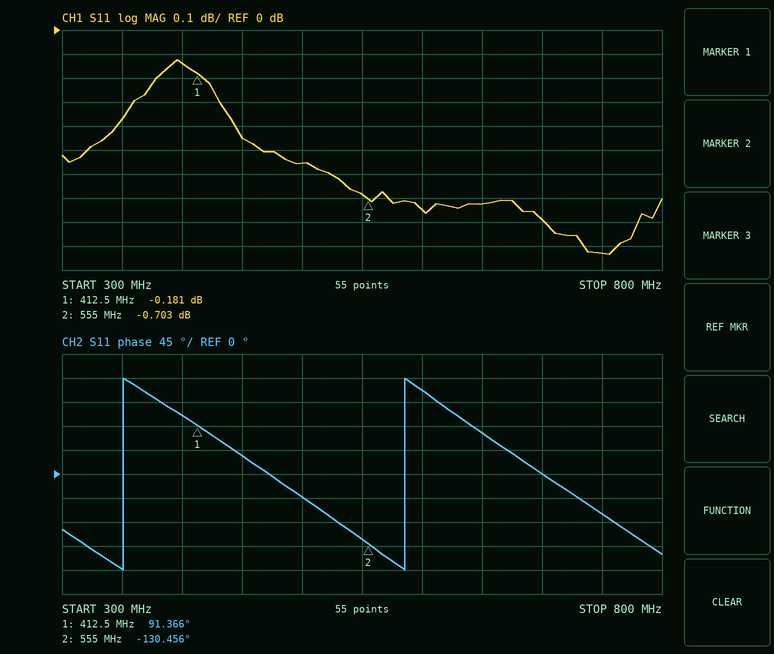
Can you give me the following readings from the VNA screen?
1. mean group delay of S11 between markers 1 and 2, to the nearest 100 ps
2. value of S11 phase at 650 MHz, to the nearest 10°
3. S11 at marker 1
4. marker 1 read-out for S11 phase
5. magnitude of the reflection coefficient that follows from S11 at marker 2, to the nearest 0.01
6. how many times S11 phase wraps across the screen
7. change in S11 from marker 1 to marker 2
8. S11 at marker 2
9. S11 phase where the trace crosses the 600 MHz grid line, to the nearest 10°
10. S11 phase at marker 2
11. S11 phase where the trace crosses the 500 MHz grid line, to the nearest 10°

4.3 ns
80°
-0.181 dB
91.366°
0.92
2
-0.522 dB
-0.703 dB
160°
-130.456°
-40°
